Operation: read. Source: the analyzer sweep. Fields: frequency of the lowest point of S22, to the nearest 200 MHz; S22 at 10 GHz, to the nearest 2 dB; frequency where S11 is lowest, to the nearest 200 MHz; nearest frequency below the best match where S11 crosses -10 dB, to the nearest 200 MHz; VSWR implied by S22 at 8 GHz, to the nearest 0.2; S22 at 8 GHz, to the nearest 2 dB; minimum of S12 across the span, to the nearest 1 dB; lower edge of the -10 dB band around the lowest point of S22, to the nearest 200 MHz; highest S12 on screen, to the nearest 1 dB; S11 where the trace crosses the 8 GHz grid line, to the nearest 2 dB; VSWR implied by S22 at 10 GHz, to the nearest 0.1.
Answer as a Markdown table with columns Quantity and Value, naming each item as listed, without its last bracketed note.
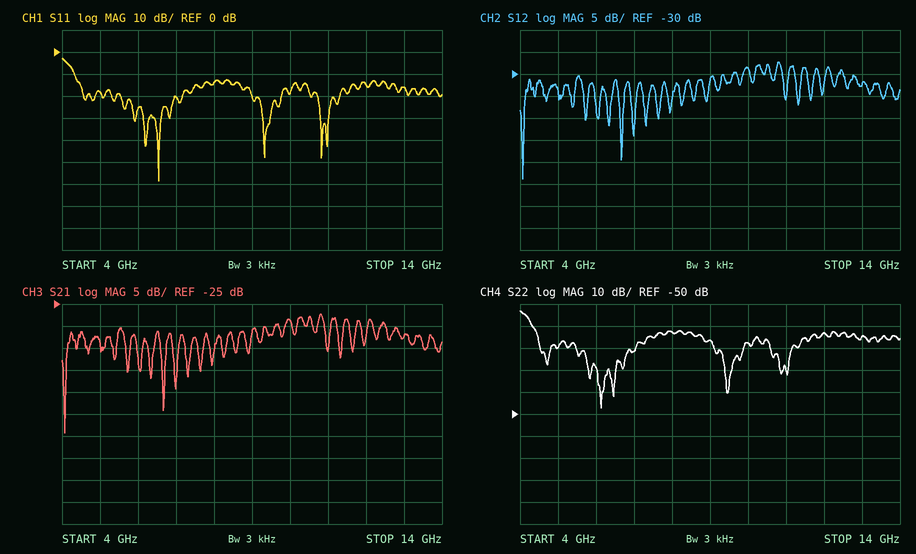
| Quantity | Value |
|---|---|
| frequency of the lowest point of S22, to the nearest 200 MHz | 6.2 GHz |
| S22 at 10 GHz, to the nearest 2 dB | -18 dB |
| frequency where S11 is lowest, to the nearest 200 MHz | 6.6 GHz |
| nearest frequency below the best match where S11 crosses -10 dB, to the nearest 200 MHz | 4.4 GHz |
| VSWR implied by S22 at 8 GHz, to the nearest 0.2 | 1.6 |
| S22 at 8 GHz, to the nearest 2 dB | -12 dB |
| minimum of S12 across the span, to the nearest 1 dB | -54 dB |
| lower edge of the -10 dB band around the lowest point of S22, to the nearest 200 MHz | 4.4 GHz |
| highest S12 on screen, to the nearest 1 dB | -27 dB |
| S11 where the trace crosses the 8 GHz grid line, to the nearest 2 dB | -14 dB |
| VSWR implied by S22 at 10 GHz, to the nearest 0.1 | 1.3 |
